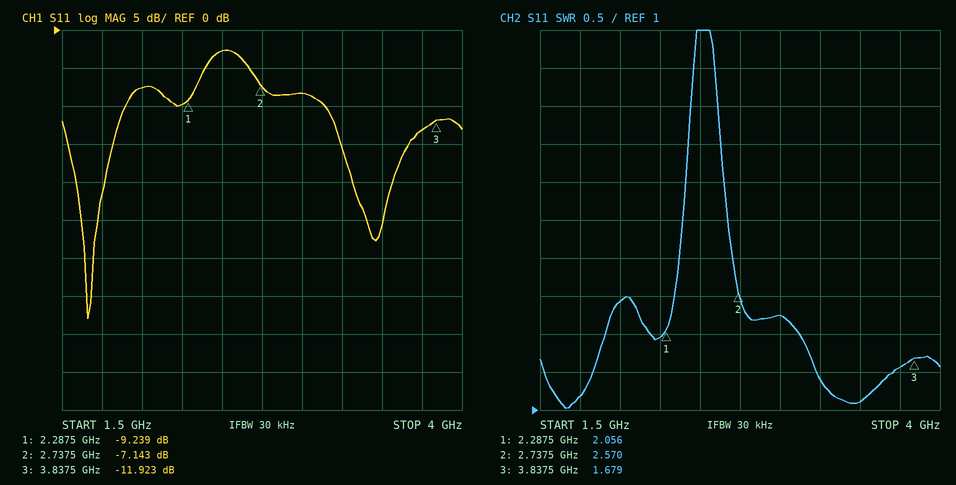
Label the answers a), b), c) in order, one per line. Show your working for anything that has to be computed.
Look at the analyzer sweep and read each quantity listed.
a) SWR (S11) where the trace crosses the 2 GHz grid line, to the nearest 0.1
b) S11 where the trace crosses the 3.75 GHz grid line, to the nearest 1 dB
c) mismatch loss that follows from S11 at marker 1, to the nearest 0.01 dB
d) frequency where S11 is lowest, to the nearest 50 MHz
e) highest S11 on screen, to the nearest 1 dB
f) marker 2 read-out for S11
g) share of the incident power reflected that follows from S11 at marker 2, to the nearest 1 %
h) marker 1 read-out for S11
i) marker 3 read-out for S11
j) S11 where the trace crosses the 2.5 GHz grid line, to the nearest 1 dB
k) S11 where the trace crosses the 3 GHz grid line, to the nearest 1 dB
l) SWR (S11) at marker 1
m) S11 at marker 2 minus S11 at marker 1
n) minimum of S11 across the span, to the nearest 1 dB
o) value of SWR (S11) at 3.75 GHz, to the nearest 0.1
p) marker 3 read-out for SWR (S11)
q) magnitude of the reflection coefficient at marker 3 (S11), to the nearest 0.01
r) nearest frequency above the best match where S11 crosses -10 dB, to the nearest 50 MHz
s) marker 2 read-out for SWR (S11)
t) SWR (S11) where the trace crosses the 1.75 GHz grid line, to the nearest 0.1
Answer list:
a) 2.4
b) -13 dB
c) −10 log10(1 − 10^(-9.239/10)) ≈ 0.55 dB
d) 1.65 GHz
e) -3 dB
f) -7.143 dB
g) 10^(-7.143/10) ≈ 19 %
h) -9.239 dB
i) -11.923 dB
j) -3 dB
k) -8 dB
l) 2.056
m) -7.143 − (-9.239) = 2.096 dB
n) -38 dB
o) 1.6
p) 1.679
q) 10^(-11.923/20) ≈ 0.25
r) 1.90 GHz
s) 2.570
t) 1.2
